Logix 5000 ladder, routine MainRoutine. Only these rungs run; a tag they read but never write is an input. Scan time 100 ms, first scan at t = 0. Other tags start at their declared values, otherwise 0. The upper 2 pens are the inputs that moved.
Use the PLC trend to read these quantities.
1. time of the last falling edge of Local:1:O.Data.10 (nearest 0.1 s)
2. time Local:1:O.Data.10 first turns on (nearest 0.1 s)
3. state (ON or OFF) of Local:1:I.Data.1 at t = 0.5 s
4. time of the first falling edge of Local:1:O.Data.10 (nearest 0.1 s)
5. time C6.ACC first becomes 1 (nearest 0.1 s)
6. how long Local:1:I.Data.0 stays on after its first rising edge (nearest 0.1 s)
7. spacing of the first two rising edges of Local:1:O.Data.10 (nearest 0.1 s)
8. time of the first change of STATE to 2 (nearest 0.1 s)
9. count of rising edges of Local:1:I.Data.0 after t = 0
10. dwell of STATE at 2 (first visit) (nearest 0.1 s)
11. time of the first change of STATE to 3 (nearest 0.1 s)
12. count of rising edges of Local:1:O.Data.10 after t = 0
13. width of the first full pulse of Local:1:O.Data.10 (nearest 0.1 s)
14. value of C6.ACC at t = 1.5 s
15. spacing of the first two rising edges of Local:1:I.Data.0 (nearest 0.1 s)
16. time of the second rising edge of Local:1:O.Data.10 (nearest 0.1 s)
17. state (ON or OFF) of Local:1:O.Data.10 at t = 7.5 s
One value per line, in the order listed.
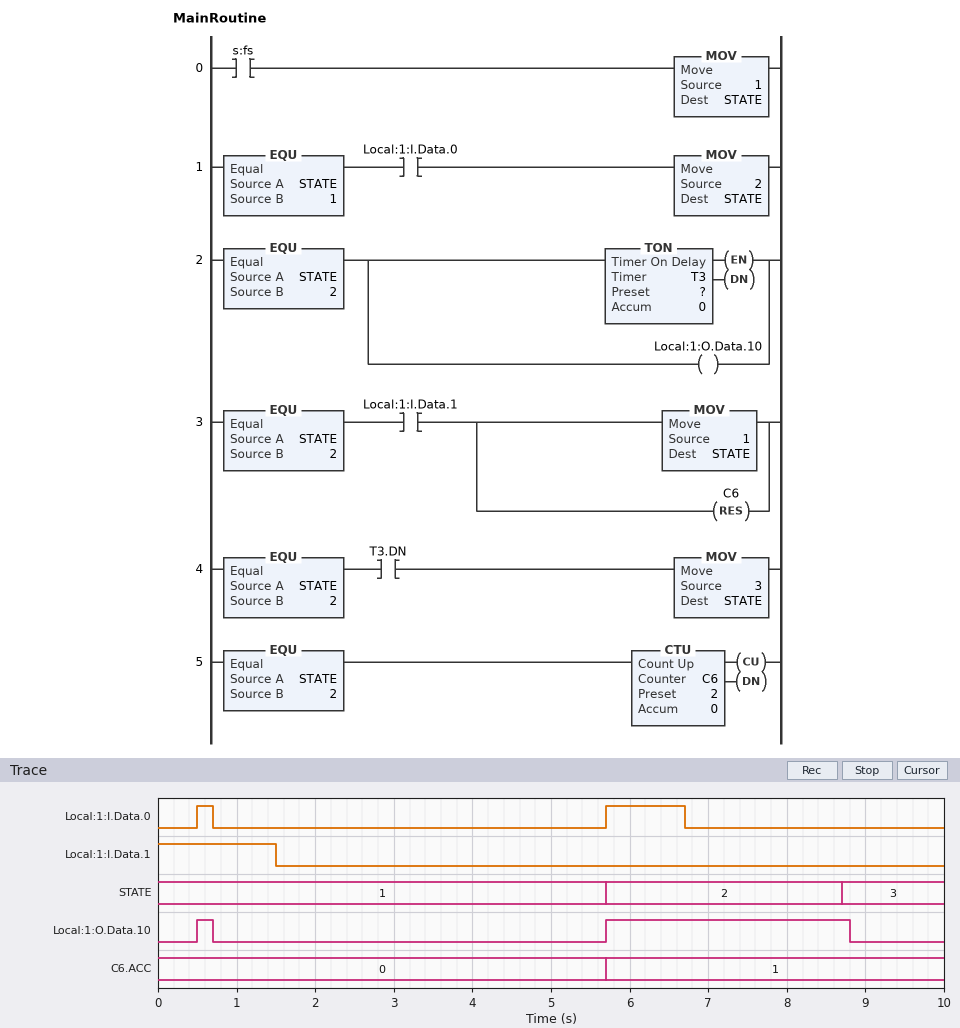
8.8 s
0.5 s
ON
0.7 s
5.7 s
0.2 s
5.2 s
5.7 s
2
3.0 s
8.7 s
2
0.2 s
0
5.2 s
5.7 s
ON
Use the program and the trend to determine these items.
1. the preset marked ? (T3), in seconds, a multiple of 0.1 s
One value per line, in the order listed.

3.0 s
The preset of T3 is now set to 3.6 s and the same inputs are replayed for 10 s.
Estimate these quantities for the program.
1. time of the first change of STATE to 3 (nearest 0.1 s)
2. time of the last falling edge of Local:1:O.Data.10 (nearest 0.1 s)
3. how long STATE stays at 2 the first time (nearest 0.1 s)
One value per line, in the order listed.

9.3 s
9.4 s
3.6 s
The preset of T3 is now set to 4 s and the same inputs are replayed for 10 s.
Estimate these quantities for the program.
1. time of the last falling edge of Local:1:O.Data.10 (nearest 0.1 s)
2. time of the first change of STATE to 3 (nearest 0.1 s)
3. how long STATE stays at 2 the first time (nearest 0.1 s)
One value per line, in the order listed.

9.8 s
9.7 s
4.0 s
